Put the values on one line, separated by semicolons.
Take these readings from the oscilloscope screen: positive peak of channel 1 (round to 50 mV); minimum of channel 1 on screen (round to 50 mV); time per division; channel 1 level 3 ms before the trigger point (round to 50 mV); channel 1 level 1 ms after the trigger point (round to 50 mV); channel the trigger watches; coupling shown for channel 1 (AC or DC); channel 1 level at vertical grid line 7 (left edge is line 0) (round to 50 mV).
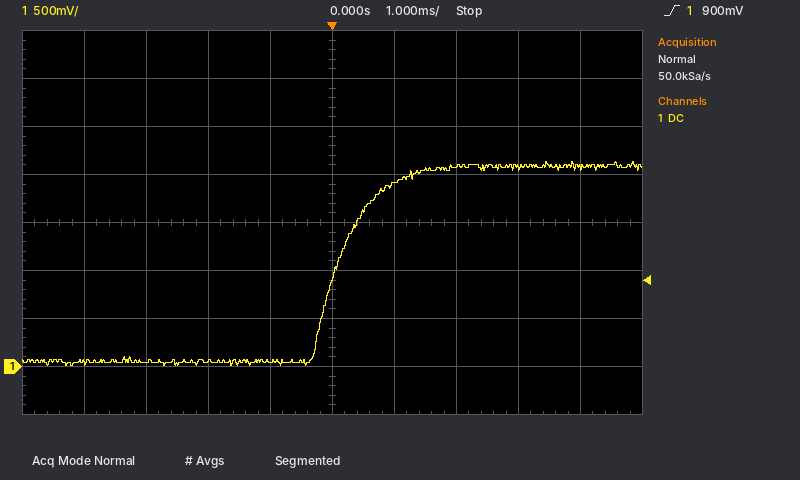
2.15 V; 0 mV; 1 ms; 50 mV; 1.90 V; channel 1; DC; 2.10 V
